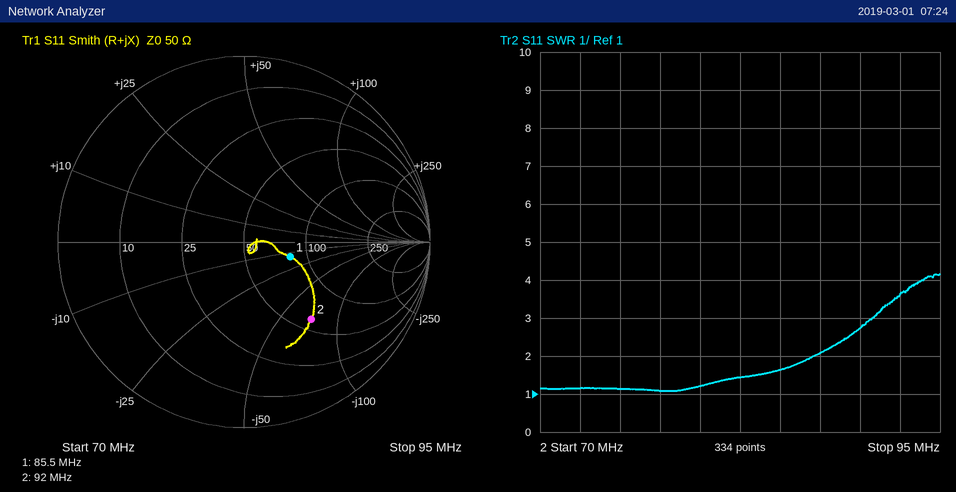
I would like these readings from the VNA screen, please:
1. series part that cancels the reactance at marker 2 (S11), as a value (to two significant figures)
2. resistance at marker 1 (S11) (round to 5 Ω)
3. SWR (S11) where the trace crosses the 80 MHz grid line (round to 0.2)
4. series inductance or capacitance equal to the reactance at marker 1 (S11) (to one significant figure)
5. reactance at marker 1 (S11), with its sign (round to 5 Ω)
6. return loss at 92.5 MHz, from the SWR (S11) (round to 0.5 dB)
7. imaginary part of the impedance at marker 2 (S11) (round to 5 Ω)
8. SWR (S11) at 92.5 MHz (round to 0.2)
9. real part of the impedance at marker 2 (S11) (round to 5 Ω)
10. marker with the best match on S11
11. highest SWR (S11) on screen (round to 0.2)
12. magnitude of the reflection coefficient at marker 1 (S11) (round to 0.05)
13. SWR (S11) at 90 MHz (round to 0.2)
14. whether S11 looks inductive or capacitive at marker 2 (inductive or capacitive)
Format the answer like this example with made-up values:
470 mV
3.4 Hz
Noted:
120 nH
80 Ω
1.2
100 pF
-15 Ω
5.0 dB
-70 Ω
3.6
60 Ω
marker 1
4.2
0.25
2.8
capacitive
